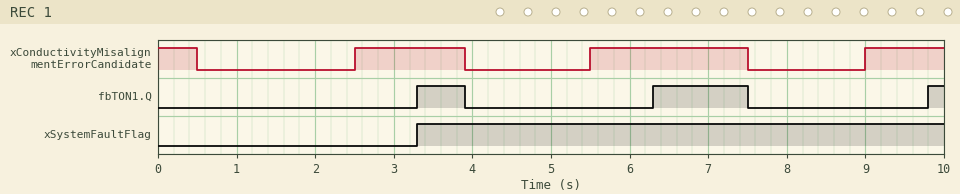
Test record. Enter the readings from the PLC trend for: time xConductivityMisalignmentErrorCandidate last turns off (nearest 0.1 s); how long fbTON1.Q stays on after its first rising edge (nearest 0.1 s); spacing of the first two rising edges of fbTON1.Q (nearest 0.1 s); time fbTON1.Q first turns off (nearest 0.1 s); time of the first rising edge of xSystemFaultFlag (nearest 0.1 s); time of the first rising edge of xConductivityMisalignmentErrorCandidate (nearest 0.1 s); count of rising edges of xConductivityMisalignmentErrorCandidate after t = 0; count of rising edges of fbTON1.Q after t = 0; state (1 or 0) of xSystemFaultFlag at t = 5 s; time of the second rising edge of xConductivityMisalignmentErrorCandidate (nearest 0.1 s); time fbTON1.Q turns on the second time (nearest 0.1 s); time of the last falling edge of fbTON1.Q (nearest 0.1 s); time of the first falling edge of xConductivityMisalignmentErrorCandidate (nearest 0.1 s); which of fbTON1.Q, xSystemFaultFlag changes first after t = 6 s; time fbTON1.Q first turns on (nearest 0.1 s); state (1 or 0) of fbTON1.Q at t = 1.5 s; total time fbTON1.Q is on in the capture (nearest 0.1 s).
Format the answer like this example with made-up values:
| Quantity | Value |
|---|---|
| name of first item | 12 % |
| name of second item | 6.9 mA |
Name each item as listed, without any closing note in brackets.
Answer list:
| Quantity | Value |
|---|---|
| time xConductivityMisalignmentErrorCandidate last turns off | 7.5 s |
| how long fbTON1.Q stays on after its first rising edge | 0.6 s |
| spacing of the first two rising edges of fbTON1.Q | 3.0 s |
| time fbTON1.Q first turns off | 3.9 s |
| time of the first rising edge of xSystemFaultFlag | 3.3 s |
| time of the first rising edge of xConductivityMisalignmentErrorCandidate | 2.5 s |
| count of rising edges of xConductivityMisalignmentErrorCandidate after t = 0 | 3 |
| count of rising edges of fbTON1.Q after t = 0 | 3 |
| state (1 or 0) of xSystemFaultFlag at t = 5 s | 1 |
| time of the second rising edge of xConductivityMisalignmentErrorCandidate | 5.5 s |
| time fbTON1.Q turns on the second time | 6.3 s |
| time of the last falling edge of fbTON1.Q | 7.5 s |
| time of the first falling edge of xConductivityMisalignmentErrorCandidate | 0.5 s |
| which of fbTON1.Q, xSystemFaultFlag changes first after t = 6 s | fbTON1.Q |
| time fbTON1.Q first turns on | 3.3 s |
| state (1 or 0) of fbTON1.Q at t = 1.5 s | 0 |
| total time fbTON1.Q is on in the capture | 2.0 s |
